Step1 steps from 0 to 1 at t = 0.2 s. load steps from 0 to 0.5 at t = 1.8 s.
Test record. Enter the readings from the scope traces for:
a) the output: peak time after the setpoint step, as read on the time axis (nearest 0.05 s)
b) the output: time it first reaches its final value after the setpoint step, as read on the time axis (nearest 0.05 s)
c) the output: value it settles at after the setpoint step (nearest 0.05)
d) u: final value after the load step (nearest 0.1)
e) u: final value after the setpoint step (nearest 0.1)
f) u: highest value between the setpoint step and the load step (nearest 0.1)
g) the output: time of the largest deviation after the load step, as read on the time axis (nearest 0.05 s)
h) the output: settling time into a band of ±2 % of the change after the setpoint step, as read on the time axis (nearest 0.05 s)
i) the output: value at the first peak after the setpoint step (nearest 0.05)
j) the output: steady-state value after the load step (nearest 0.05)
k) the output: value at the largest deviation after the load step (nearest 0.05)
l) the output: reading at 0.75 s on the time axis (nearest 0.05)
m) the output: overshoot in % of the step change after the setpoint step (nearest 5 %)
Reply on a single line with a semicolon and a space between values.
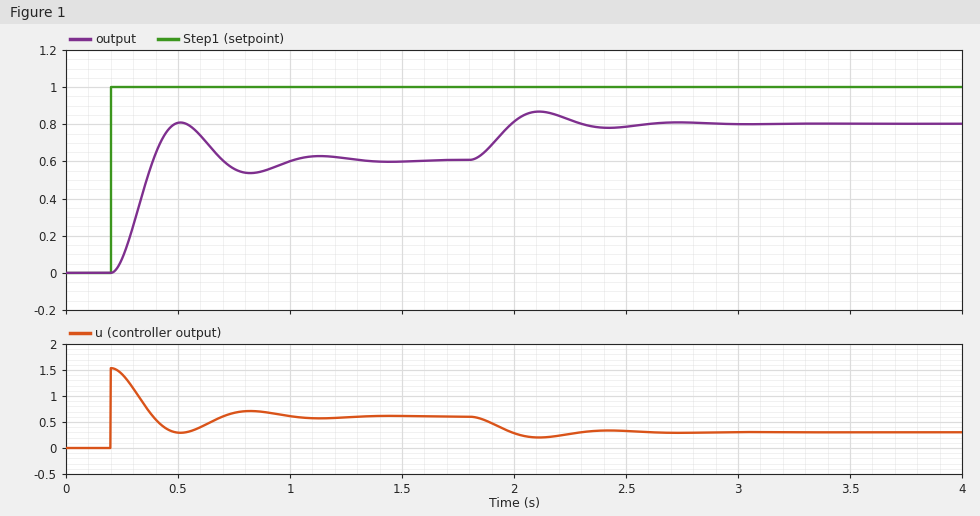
0.50 s; 0.40 s; 0.60; 0.3; 0.6; 1.5; 2.10 s; 1.25 s; 0.80; 0.80; 0.85; 0.55; 35 %
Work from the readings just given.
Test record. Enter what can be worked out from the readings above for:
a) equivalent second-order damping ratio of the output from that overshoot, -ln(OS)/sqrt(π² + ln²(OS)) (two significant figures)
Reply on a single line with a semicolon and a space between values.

0.32
